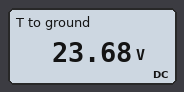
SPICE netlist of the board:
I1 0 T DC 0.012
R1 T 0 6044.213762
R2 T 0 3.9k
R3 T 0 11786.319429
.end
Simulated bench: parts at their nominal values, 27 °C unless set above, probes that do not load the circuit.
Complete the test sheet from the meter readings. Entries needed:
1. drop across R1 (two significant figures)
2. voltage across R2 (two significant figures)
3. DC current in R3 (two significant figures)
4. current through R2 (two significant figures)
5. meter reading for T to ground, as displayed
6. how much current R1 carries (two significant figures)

24 V
24 V
2.0 mA
6.1 mA
23.68 V
3.9 mA
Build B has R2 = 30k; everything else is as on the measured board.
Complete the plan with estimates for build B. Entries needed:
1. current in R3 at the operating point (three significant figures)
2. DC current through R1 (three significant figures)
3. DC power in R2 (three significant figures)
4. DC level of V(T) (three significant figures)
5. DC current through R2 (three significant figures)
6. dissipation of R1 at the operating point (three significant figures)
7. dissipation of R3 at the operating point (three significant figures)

3.59 mA
7.00 mA
59.7 mW
42.3 V
1.41 mA
296 mW
152 mW
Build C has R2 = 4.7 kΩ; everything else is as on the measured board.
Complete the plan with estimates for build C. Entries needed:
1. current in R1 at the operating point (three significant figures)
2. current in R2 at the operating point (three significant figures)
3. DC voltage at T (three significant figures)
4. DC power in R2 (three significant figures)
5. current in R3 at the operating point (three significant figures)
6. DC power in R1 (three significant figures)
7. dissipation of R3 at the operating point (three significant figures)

4.29 mA
5.51 mA
25.9 V
143 mW
2.20 mA
111 mW
57.0 mW
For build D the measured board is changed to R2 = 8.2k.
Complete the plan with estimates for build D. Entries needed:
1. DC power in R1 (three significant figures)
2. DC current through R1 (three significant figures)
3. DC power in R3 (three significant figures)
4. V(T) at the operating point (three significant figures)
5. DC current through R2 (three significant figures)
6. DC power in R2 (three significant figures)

172 mW
5.33 mA
88.2 mW
32.2 V
3.93 mA
127 mW
